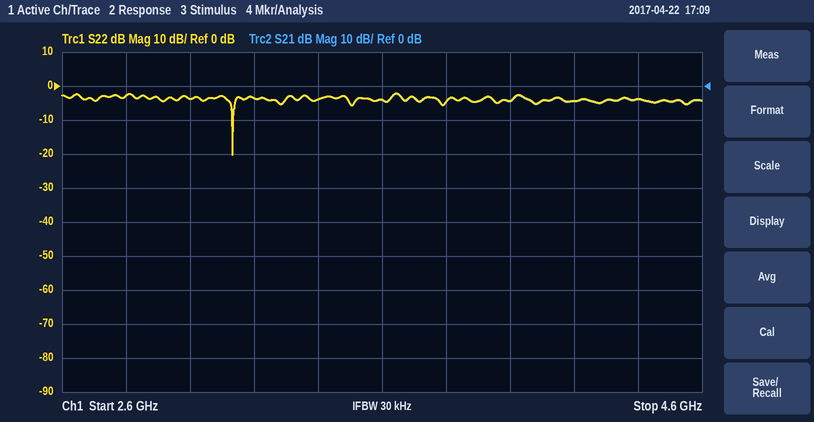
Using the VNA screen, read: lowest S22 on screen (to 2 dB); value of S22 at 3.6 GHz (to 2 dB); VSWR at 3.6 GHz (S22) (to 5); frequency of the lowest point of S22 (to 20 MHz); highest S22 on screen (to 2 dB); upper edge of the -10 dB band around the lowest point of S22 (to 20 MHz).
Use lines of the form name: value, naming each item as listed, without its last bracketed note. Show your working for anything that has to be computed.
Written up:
lowest S22 on screen: -20 dB
value of S22 at 3.6 GHz: -4 dB
VSWR at 3.6 GHz (S22): |Γ| = 10^(-4/20) = 0.6310; VSWR = (1 + 0.6310)/(1 − 0.6310) ≈ 4.42, so 5 to the nearest 5
frequency of the lowest point of S22: 3.14 GHz
highest S22 on screen: -2 dB
upper edge of the -10 dB band around the lowest point of S22: 3.14 GHz
